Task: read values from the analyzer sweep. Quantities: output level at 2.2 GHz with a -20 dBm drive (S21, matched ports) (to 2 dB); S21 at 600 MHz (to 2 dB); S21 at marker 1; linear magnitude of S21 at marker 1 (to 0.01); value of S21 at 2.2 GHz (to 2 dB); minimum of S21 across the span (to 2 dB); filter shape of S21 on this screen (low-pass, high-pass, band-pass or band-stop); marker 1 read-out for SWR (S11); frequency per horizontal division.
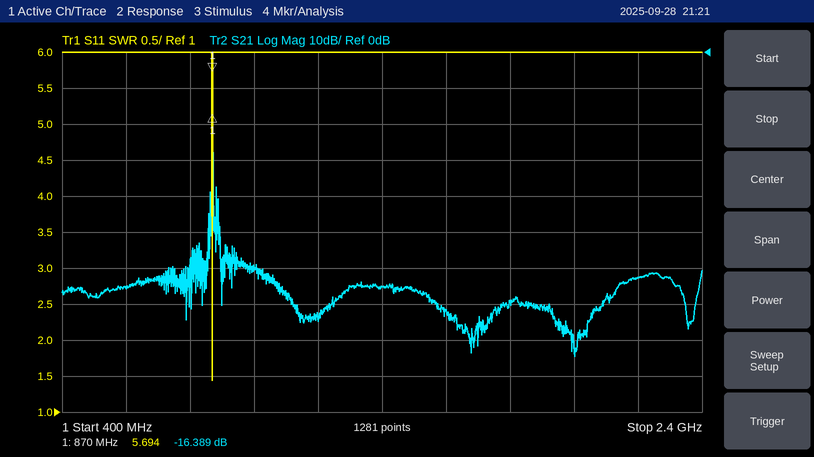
-82 dBm
-66 dB
-16.389 dB
0.15
-62 dB
-84 dB
band-pass
5.694
200 MHz
